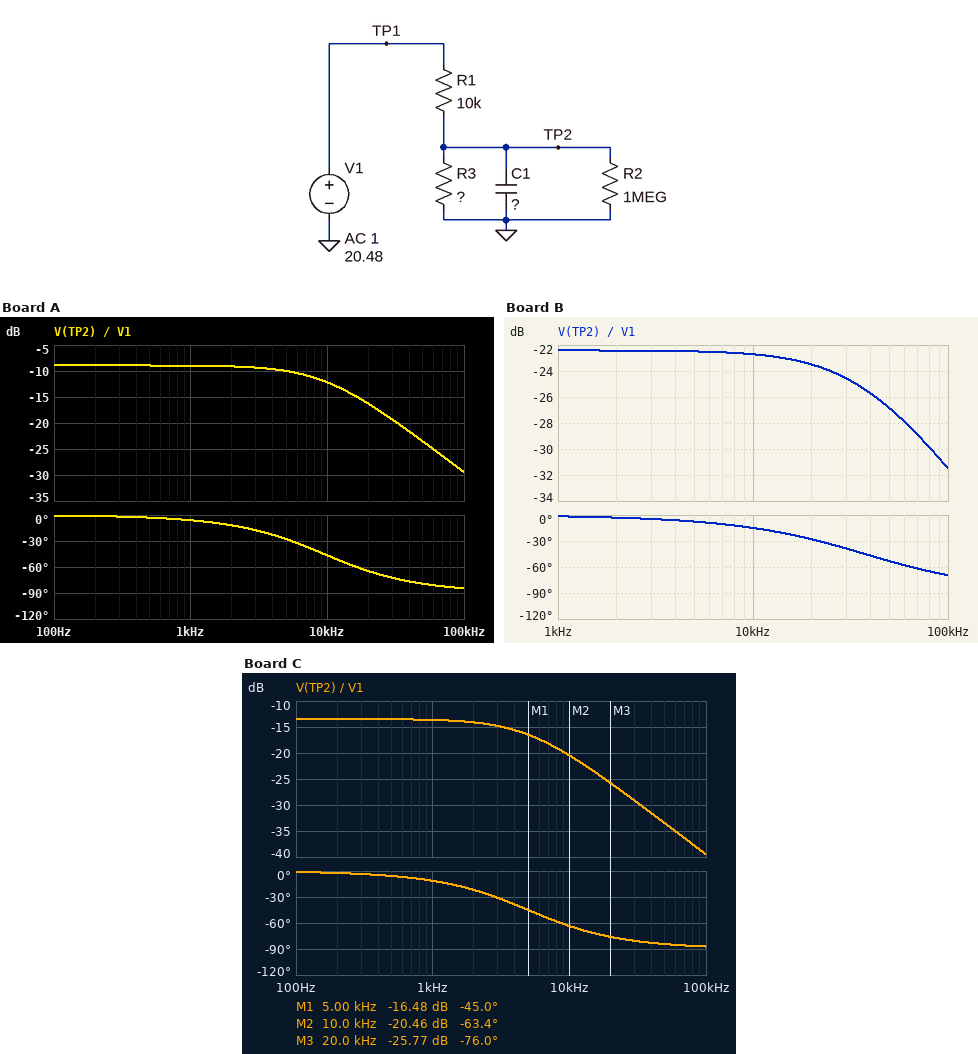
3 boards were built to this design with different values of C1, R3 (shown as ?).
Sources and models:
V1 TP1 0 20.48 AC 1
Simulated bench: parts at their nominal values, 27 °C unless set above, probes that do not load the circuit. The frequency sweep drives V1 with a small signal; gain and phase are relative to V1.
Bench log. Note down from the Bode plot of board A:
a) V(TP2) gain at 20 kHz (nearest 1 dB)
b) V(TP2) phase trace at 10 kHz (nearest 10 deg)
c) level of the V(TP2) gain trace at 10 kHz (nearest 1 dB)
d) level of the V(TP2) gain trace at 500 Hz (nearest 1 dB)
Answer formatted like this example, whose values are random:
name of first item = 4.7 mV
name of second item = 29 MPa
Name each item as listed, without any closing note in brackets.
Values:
V(TP2) gain at 20 kHz = -16 dB
V(TP2) phase trace at 10 kHz = -50 deg
level of the V(TP2) gain trace at 10 kHz = -12 dB
level of the V(TP2) gain trace at 500 Hz = -9 dB
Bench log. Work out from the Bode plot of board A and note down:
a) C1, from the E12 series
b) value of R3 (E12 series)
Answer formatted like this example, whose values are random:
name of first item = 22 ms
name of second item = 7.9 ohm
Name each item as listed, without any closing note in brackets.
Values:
C1, from the E12 series = 4.7 nF
value of R3 = 5.6 kΩ
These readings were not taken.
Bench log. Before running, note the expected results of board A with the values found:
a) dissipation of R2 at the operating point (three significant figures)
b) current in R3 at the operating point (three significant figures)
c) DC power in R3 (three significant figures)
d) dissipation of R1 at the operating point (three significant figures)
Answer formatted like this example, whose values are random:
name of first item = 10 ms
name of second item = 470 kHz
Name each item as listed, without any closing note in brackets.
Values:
dissipation of R2 at the operating point = 53.7 µW
current in R3 at the operating point = 1.31 mA
DC power in R3 = 9.58 mW
dissipation of R1 at the operating point = 17.3 mW
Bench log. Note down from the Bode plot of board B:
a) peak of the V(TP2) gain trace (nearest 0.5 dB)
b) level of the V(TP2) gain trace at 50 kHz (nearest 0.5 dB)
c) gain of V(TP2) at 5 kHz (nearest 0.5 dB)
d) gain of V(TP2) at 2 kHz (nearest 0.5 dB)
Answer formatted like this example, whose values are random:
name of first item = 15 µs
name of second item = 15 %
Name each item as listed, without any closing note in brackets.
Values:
peak of the V(TP2) gain trace = -22.5 dB
level of the V(TP2) gain trace at 50 kHz = -27.0 dB
gain of V(TP2) at 5 kHz = -22.5 dB
gain of V(TP2) at 2 kHz = -22.5 dB
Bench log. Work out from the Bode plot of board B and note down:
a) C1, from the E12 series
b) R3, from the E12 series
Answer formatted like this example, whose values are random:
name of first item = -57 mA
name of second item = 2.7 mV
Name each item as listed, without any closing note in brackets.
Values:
C1, from the E12 series = 5.6 nF
R3, from the E12 series = 820 Ω
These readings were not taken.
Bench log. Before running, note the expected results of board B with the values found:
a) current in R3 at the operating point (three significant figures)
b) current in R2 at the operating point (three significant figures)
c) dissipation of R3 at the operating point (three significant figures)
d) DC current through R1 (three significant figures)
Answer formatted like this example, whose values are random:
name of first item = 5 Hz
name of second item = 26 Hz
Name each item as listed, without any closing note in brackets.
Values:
current in R3 at the operating point = 1.89 mA
current in R2 at the operating point = 1.55 µA
dissipation of R3 at the operating point = 2.93 mW
DC current through R1 = 1.89 mA
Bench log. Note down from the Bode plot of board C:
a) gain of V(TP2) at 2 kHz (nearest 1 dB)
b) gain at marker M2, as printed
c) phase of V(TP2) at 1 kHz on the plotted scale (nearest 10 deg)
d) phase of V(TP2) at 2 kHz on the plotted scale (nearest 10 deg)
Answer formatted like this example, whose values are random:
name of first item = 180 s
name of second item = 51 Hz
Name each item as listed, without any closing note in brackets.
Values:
gain of V(TP2) at 2 kHz = -14 dB
gain at marker M2, as printed = -20.46 dB
phase of V(TP2) at 1 kHz on the plotted scale = -10 deg
phase of V(TP2) at 2 kHz on the plotted scale = -20 deg
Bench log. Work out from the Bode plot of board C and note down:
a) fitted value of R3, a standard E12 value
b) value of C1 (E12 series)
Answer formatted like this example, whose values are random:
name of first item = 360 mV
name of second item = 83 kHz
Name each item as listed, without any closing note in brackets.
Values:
fitted value of R3, a standard E12 value = 2.7 kΩ
value of C1 = 15 nF
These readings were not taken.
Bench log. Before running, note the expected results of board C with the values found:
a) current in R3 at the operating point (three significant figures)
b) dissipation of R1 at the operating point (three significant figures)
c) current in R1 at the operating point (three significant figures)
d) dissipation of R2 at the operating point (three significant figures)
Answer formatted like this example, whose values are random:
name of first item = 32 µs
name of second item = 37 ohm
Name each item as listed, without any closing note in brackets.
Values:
current in R3 at the operating point = 1.61 mA
dissipation of R1 at the operating point = 26.0 mW
current in R1 at the operating point = 1.61 mA
dissipation of R2 at the operating point = 18.9 µW
